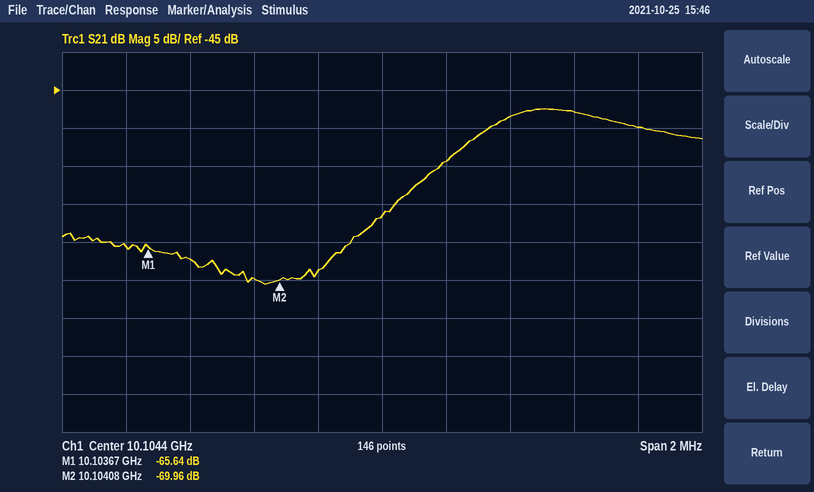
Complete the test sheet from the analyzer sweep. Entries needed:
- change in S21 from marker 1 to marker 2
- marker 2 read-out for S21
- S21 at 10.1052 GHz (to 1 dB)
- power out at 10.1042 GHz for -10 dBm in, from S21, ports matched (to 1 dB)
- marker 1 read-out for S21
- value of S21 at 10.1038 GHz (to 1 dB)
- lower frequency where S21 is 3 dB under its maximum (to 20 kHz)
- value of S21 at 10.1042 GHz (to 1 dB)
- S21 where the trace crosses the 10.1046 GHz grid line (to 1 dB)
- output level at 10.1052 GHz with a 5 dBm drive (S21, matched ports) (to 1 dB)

-4.32 dB
-69.96 dB
-50 dB
-79 dBm
-65.64 dB
-67 dB
10.10472 GHz
-69 dB
-54 dB
-45 dBm
